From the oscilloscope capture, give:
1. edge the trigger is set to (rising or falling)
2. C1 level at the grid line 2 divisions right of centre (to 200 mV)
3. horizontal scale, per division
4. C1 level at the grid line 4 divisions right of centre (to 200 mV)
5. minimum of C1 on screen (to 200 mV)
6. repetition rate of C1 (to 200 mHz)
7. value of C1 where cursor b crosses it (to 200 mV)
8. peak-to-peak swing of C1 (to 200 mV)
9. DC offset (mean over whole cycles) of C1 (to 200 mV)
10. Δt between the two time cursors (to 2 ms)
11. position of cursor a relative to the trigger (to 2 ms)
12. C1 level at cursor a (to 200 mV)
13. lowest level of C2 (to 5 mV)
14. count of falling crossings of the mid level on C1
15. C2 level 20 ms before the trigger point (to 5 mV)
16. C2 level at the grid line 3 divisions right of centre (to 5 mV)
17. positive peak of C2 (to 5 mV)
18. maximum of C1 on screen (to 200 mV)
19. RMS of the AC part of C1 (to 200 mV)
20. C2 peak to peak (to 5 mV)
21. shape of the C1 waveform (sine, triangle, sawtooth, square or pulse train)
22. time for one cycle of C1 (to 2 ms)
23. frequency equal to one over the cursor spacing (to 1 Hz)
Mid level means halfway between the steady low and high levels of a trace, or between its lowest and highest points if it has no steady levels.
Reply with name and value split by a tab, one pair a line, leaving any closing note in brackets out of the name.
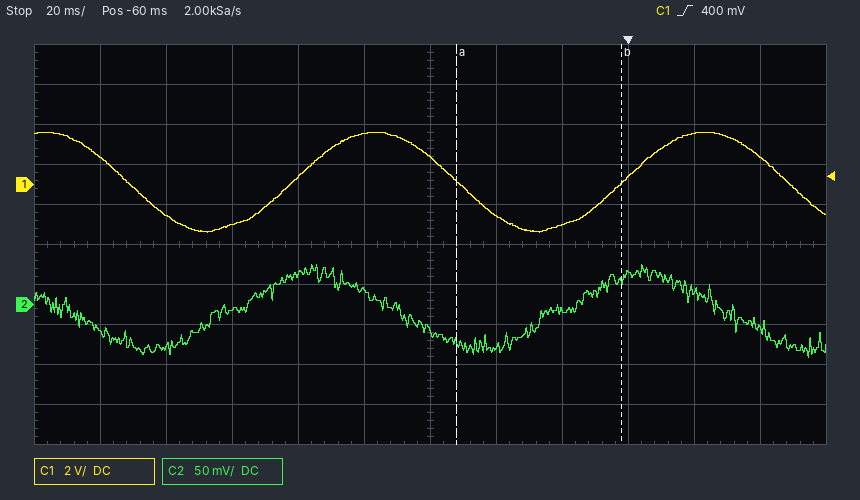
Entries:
edge the trigger is set to	rising
C1 level at the grid line 2 divisions right of centre	-2.0 V
horizontal scale, per division	20 ms
C1 level at the grid line 4 divisions right of centre	2.6 V
minimum of C1 on screen	-2.4 V
repetition rate of C1	10.0 Hz
value of C1 where cursor b crosses it	0.0 V
peak-to-peak swing of C1	5.0 V
DC offset (mean over whole cycles) of C1	200 mV
Δt between the two time cursors	50 ms
position of cursor a relative to the trigger	-52 ms
C1 level at cursor a	200 mV
lowest level of C2	-65 mV
count of falling crossings of the mid level on C1	3
C2 level 20 ms before the trigger point	-10 mV
C2 level at the grid line 3 divisions right of centre	40 mV
positive peak of C2	50 mV
maximum of C1 on screen	2.6 V
RMS of the AC part of C1	1.8 V
C2 peak to peak	115 mV
shape of the C1 waveform	sine
time for one cycle of C1	100 ms
frequency equal to one over the cursor spacing	20 Hz
